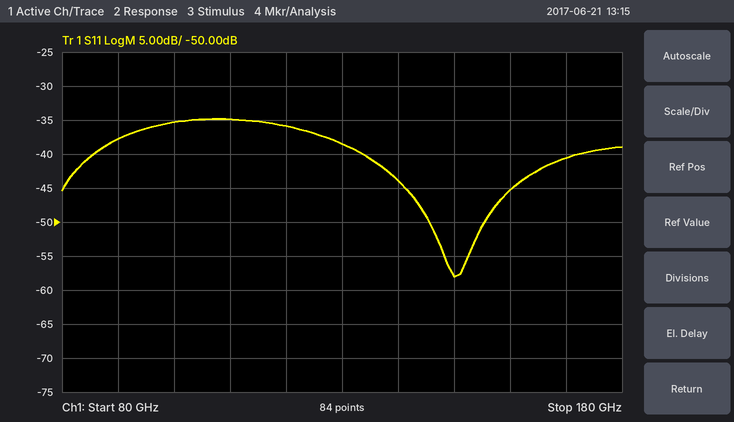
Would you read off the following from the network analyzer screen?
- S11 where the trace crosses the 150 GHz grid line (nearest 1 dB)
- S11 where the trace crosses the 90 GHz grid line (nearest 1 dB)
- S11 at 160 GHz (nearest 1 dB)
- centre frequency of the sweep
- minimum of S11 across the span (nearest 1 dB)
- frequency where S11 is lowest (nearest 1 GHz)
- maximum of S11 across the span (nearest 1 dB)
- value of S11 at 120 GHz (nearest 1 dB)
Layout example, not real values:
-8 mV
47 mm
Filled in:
-58 dB
-38 dB
-45 dB
130 GHz
-58 dB
150 GHz
-35 dB
-36 dB
